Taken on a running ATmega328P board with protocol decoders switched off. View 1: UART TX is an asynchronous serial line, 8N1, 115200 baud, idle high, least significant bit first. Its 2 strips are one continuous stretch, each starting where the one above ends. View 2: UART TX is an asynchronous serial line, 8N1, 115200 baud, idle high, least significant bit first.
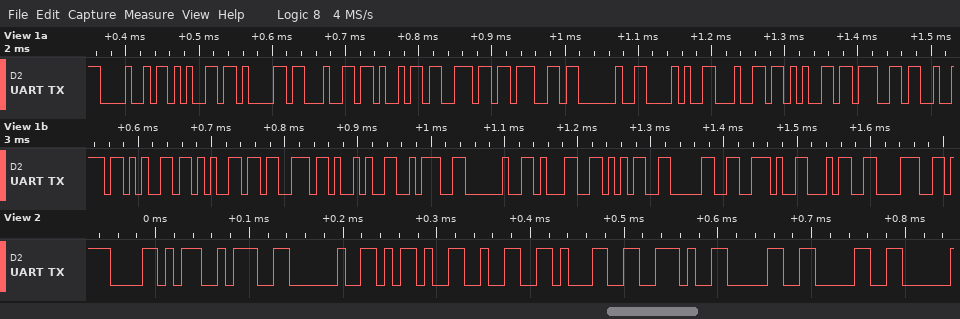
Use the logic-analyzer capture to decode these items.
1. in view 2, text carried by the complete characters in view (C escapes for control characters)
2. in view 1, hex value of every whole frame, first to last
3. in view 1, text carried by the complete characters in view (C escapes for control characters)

"X: -21.00"
48 65 61 64 69 6E 67 20 28 64 65 67 72 65 65 73 29 3A 20 31 35 30 2E 34 38
"Heading (degrees): 150.48"
